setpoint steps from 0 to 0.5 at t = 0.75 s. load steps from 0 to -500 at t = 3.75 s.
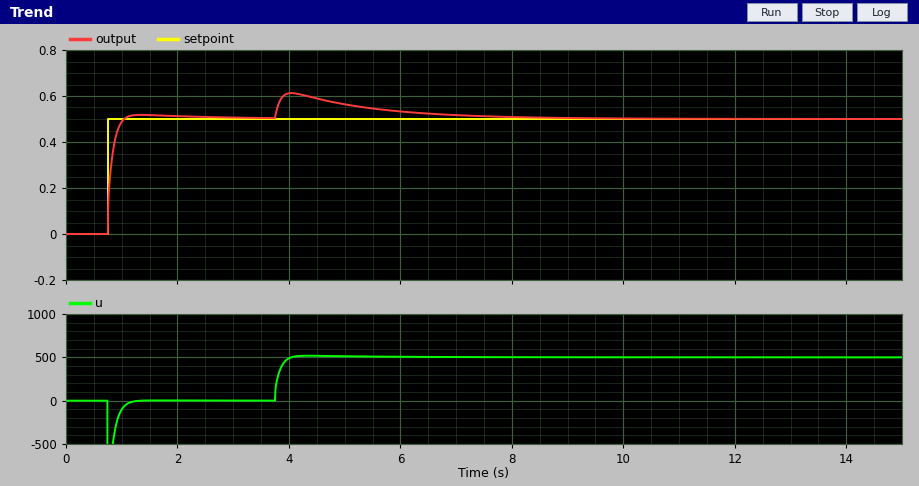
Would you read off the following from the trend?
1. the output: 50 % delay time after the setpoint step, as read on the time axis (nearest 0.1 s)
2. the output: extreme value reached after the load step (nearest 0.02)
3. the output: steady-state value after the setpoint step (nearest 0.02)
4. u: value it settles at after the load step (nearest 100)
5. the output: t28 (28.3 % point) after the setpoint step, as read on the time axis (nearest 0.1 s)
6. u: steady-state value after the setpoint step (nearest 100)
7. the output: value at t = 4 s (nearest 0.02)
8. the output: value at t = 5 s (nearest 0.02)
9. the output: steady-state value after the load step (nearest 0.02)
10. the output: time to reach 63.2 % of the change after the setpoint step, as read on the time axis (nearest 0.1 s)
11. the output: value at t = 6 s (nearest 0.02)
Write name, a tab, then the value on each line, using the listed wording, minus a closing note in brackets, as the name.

the output: 50 % delay time after the setpoint step, as read on the time axis	0.8 s
the output: extreme value reached after the load step	0.62
the output: steady-state value after the setpoint step	0.50
u: value it settles at after the load step	500
the output: t28 (28.3 % point) after the setpoint step, as read on the time axis	0.8 s
u: steady-state value after the setpoint step	0
the output: value at t = 4 s	0.62
the output: value at t = 5 s	0.56
the output: steady-state value after the load step	0.50
the output: time to reach 63.2 % of the change after the setpoint step, as read on the time axis	0.8 s
the output: value at t = 6 s	0.54
